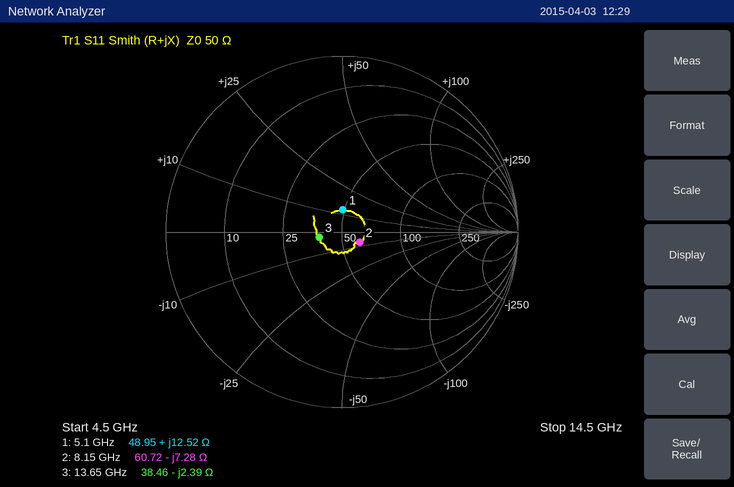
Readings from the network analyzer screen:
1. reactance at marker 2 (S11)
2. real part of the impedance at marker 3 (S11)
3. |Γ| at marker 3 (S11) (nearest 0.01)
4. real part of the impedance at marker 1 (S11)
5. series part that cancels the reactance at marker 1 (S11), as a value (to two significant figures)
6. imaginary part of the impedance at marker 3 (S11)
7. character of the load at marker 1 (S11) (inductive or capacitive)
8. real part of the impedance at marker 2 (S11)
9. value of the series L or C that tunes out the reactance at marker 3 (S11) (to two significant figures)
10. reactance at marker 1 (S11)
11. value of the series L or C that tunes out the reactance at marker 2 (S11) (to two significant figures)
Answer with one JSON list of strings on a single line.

["-7.28 Ω", "38.46 Ω", "0.13", "48.95 Ω", "2.5 pF", "-2.39 Ω", "inductive", "60.72 Ω", "28 pH", "+12.52 Ω", "140 pH"]
